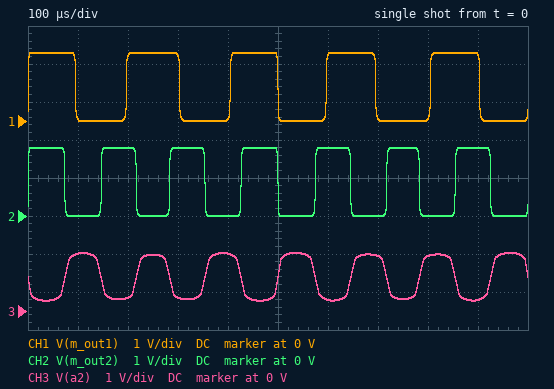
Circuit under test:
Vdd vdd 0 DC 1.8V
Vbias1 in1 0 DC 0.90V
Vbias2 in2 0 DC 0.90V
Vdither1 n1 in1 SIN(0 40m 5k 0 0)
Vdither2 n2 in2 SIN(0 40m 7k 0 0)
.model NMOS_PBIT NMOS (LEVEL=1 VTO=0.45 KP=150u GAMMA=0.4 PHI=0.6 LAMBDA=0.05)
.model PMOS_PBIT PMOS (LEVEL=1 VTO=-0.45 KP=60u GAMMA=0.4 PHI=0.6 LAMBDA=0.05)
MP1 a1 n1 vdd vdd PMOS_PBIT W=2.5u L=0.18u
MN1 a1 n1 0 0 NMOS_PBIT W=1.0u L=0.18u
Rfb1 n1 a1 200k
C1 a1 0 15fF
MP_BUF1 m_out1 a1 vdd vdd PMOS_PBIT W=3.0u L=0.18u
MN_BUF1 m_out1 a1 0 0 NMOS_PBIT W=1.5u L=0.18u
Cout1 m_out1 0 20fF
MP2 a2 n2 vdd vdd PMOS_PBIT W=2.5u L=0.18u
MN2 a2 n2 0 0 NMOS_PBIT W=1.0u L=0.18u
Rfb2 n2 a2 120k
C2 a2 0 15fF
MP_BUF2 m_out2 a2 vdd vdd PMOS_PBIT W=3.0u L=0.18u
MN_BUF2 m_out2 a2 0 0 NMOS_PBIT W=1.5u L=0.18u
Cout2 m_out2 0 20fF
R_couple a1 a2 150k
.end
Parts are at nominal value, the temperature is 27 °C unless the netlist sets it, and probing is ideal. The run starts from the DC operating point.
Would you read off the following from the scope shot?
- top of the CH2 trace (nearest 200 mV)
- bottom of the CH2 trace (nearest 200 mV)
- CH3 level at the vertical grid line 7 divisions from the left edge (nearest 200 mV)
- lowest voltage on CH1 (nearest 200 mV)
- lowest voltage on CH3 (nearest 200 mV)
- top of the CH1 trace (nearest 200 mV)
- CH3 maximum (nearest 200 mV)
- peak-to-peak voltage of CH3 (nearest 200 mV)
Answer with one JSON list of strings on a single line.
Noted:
["1.8 V", "0 V", "1.4 V", "0 V", "200 mV", "1.8 V", "1.6 V", "1.2 V"]
